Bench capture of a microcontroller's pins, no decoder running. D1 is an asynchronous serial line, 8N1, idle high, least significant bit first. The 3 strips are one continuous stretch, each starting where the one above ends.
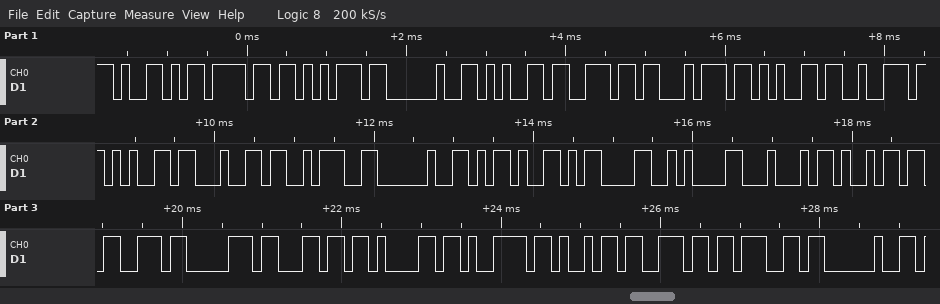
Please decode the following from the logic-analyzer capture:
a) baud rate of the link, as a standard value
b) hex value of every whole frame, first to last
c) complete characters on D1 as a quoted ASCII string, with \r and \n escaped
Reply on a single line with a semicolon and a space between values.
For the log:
9600 baud; 59 6F 75 20 65 6E 74 65 72 65 64 3A 20 2D 0D 0A 44 69 73 70 6C 61 79 69 6E 67 20; "You entered: -\r\nDisplaying "
